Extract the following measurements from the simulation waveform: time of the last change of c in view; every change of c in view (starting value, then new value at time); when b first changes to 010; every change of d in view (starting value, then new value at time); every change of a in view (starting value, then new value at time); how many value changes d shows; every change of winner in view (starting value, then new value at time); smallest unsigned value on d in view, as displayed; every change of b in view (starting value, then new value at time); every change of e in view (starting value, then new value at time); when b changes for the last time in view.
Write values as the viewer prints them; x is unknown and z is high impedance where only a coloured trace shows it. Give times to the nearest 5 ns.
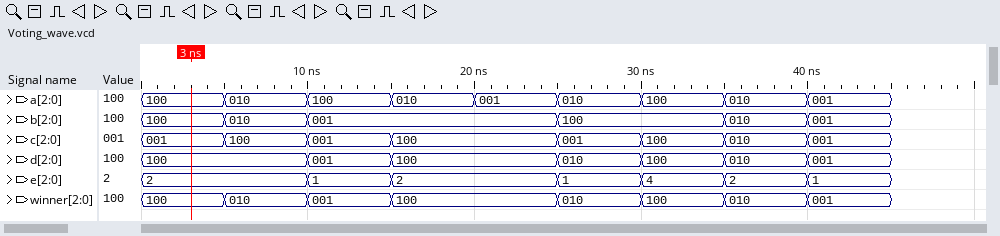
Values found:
40 ns
001, 100 at 5 ns, 001 at 10 ns, 100 at 15 ns, 001 at 25 ns, 100 at 30 ns, 010 at 35 ns, 001 at 40 ns
5 ns
100, 001 at 10 ns, 100 at 15 ns, 010 at 25 ns, 100 at 30 ns, 010 at 35 ns, 001 at 40 ns
100, 010 at 5 ns, 100 at 10 ns, 010 at 15 ns, 001 at 20 ns, 010 at 25 ns, 100 at 30 ns, 010 at 35 ns, 001 at 40 ns
6
100, 010 at 5 ns, 001 at 10 ns, 100 at 15 ns, 010 at 25 ns, 100 at 30 ns, 010 at 35 ns, 001 at 40 ns
001
100, 010 at 5 ns, 001 at 10 ns, 100 at 25 ns, 010 at 35 ns, 001 at 40 ns
2, 1 at 10 ns, 2 at 15 ns, 1 at 25 ns, 4 at 30 ns, 2 at 35 ns, 1 at 40 ns
40 ns
